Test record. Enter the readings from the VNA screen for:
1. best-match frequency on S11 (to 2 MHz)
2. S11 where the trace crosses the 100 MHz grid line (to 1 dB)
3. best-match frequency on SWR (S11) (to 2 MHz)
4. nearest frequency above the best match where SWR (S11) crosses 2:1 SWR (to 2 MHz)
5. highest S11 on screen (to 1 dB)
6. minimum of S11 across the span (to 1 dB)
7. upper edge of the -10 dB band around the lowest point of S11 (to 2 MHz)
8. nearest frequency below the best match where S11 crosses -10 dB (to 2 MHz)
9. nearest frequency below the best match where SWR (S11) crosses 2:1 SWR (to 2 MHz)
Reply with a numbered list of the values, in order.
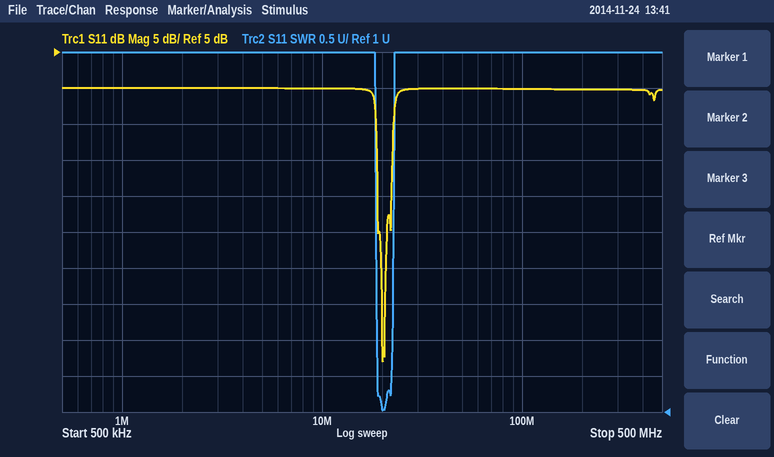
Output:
1. 20 MHz
2. 0 dB
3. 20 MHz
4. 22 MHz
5. 0 dB
6. -38 dB
7. 22 MHz
8. 18 MHz
9. 18 MHz
